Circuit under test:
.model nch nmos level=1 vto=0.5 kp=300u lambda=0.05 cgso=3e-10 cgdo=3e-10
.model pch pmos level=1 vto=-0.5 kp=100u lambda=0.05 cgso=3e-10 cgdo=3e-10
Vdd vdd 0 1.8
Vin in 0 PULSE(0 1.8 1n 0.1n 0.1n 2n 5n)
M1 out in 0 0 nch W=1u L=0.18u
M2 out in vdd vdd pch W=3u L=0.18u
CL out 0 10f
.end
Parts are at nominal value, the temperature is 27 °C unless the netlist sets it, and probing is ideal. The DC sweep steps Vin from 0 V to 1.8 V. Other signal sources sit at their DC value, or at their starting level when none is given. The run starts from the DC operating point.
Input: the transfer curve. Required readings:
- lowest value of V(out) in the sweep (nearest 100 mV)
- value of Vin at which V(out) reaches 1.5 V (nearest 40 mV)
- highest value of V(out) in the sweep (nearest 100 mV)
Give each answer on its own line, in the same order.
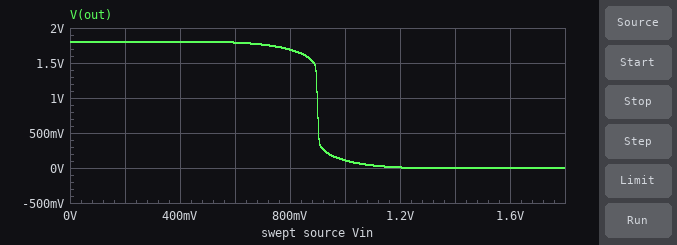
0 V
880 mV
1.8 V
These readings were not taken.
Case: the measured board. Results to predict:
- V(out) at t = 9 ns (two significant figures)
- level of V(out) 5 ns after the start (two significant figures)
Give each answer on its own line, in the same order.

1.8 V
1.8 V
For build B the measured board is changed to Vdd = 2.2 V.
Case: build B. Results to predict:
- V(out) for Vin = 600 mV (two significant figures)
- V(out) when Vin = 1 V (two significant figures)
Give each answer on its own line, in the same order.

2.2 V
2.0 V
